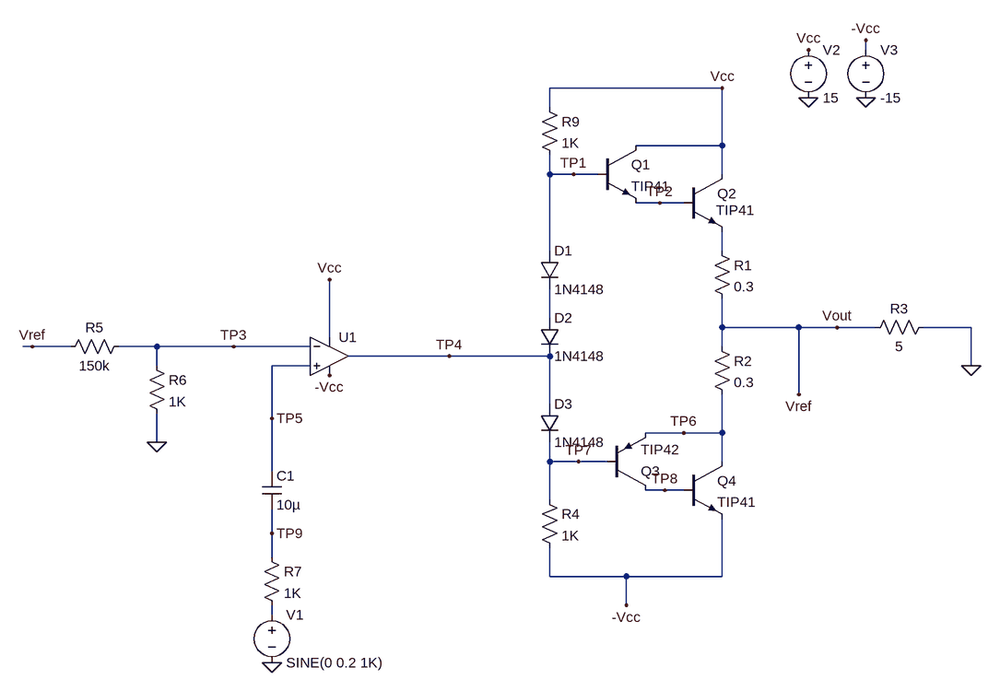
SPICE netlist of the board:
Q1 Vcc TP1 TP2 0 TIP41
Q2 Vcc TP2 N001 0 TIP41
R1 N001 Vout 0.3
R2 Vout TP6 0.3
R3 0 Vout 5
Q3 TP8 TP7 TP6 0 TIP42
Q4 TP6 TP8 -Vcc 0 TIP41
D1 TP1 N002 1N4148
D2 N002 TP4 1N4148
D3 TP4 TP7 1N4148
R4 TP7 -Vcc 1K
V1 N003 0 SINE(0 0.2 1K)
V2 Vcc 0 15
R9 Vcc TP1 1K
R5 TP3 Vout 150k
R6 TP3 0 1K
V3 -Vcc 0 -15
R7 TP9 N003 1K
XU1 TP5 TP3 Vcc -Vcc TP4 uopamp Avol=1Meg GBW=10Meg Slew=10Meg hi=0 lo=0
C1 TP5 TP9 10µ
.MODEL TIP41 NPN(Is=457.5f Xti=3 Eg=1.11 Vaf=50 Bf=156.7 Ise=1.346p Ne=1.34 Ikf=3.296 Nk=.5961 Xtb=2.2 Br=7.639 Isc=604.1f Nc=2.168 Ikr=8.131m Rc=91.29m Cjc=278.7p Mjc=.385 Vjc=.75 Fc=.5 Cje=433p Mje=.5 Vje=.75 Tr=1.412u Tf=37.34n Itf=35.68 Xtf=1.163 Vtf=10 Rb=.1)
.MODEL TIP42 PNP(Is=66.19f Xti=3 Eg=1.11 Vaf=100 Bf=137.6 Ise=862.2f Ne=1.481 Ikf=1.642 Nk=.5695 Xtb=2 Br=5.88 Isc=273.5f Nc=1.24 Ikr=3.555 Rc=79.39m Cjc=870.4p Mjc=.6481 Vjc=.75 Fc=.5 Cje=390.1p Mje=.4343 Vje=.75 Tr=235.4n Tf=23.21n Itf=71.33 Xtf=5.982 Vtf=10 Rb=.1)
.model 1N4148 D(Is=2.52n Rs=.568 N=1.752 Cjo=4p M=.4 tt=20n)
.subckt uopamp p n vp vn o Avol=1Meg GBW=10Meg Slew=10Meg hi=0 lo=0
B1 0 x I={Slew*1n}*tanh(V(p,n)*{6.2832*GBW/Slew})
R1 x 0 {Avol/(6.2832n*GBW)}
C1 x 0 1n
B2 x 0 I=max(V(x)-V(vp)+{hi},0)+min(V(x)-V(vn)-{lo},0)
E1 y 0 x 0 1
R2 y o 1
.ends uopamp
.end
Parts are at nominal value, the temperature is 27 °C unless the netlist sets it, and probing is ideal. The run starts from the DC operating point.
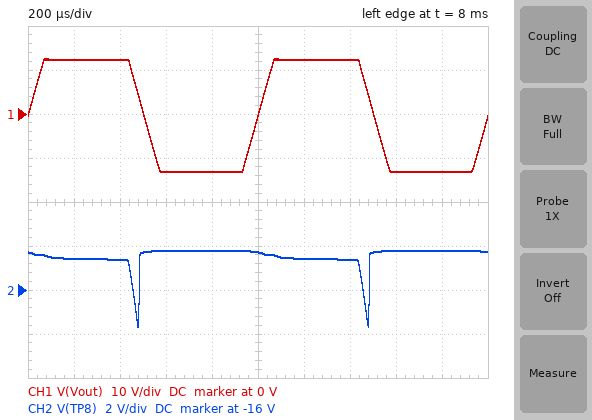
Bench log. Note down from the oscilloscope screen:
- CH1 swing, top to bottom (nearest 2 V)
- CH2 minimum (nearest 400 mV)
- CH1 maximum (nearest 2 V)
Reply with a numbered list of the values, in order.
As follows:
1. 26 V
2. -17.6 V
3. 12 V
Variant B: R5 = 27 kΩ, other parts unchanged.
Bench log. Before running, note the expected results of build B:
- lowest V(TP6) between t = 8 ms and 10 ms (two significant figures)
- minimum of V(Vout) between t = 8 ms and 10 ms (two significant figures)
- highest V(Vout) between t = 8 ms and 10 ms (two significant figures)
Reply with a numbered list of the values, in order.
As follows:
1. -5.9 V
2. -5.6 V
3. 5.6 V
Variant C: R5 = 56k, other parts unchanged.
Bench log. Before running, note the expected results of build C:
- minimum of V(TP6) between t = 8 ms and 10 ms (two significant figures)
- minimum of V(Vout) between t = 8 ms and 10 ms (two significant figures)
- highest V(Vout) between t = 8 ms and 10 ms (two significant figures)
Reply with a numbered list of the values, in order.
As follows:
1. -12 V
2. -11 V
3. 11 V
